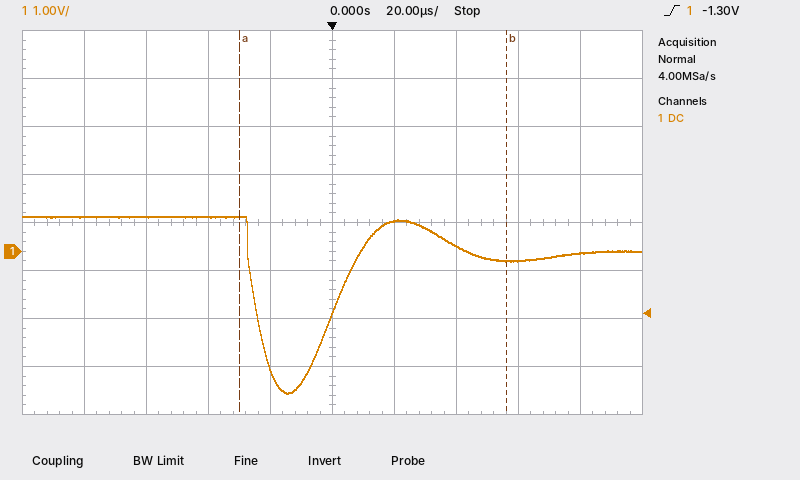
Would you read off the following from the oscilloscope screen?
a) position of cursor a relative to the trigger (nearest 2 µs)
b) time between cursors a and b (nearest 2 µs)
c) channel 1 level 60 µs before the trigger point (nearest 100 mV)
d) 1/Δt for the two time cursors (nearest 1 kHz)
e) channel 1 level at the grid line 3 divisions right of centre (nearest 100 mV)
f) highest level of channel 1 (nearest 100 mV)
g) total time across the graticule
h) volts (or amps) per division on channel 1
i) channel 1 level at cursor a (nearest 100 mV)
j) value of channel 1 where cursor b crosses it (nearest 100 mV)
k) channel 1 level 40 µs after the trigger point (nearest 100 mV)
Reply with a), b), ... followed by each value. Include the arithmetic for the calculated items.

a) -30 µs
b) 86 µs
c) 700 mV
d) 1 / 86 µs ≈ 12 kHz
e) -200 mV
f) 700 mV
g) 200 µs
h) 1 V
i) 700 mV
j) -200 mV
k) 100 mV
